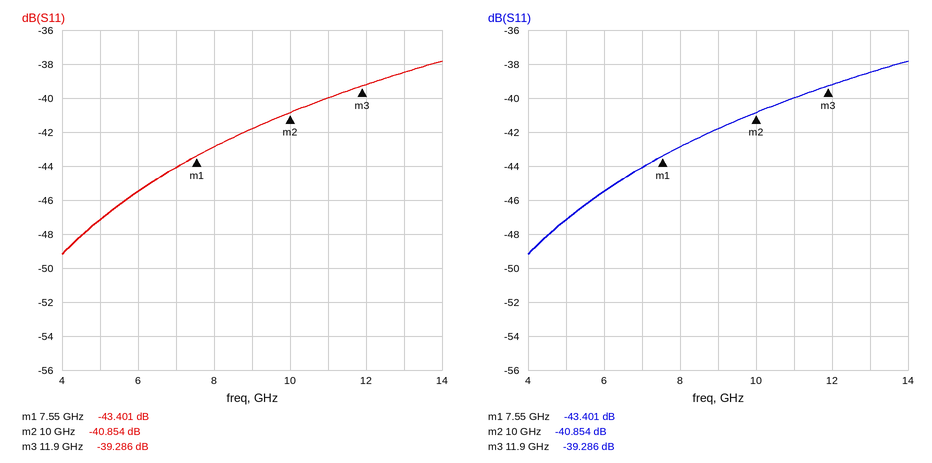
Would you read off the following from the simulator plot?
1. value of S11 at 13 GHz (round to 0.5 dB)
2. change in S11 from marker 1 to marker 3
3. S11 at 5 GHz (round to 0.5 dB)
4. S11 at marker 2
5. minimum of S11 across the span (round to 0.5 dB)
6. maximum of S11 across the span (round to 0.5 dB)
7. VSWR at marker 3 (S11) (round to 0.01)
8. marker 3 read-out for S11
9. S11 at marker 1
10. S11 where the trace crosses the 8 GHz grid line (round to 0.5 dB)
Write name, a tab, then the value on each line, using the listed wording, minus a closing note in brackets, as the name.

value of S11 at 13 GHz	-38.5 dB
change in S11 from marker 1 to marker 3	4.115 dB
S11 at 5 GHz	-47.0 dB
S11 at marker 2	-40.854 dB
minimum of S11 across the span	-49.0 dB
maximum of S11 across the span	-38.0 dB
VSWR at marker 3 (S11)	1.02
marker 3 read-out for S11	-39.286 dB
S11 at marker 1	-43.401 dB
S11 where the trace crosses the 8 GHz grid line	-43.0 dB
